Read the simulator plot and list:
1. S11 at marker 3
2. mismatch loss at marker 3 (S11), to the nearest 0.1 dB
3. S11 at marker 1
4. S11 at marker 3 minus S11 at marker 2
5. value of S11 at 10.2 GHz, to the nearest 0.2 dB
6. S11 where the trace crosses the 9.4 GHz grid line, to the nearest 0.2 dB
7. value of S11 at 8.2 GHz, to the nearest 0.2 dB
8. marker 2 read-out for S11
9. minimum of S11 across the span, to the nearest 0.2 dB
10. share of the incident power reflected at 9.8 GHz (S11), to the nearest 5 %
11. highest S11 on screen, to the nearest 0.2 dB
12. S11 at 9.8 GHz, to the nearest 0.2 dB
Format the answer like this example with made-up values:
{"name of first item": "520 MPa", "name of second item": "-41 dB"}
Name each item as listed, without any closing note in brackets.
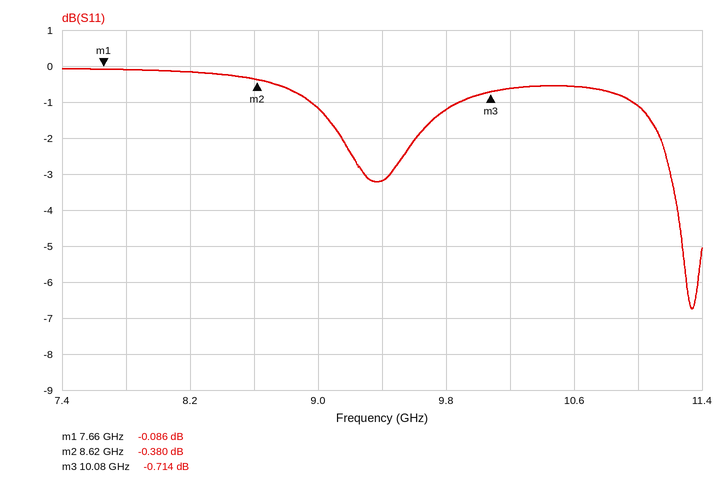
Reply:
{"S11 at marker 3": "-0.714 dB", "mismatch loss at marker 3 (S11), to the nearest 0.1 dB": "8.2 dB", "S11 at marker 1": "-0.086 dB", "S11 at marker 3 minus S11 at marker 2": "-0.334 dB", "value of S11 at 10.2 GHz, to the nearest 0.2 dB": "-0.6 dB", "S11 where the trace crosses the 9.4 GHz grid line, to the nearest 0.2 dB": "-3.2 dB", "value of S11 at 8.2 GHz, to the nearest 0.2 dB": "-0.2 dB", "marker 2 read-out for S11": "-0.380 dB", "minimum of S11 across the span, to the nearest 0.2 dB": "-6.8 dB", "share of the incident power reflected at 9.8 GHz (S11), to the nearest 5 %": "75 %", "highest S11 on screen, to the nearest 0.2 dB": "0.0 dB", "S11 at 9.8 GHz, to the nearest 0.2 dB": "-1.2 dB"}
